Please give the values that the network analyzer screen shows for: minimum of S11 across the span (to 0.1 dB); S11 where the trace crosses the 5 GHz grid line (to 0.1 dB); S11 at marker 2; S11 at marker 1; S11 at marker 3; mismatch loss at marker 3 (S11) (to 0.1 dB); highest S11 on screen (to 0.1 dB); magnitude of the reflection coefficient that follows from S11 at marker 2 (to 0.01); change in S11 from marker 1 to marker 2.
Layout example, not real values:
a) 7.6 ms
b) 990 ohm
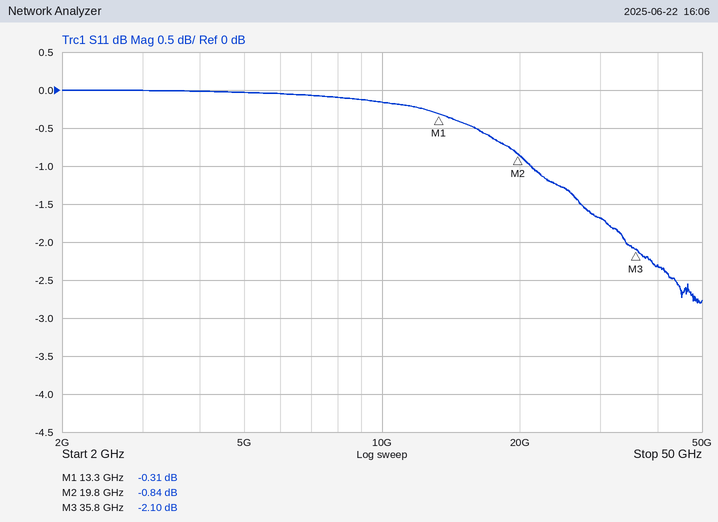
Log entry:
a) -2.8 dB
b) 0.0 dB
c) -0.84 dB
d) -0.31 dB
e) -2.10 dB
f) 4.2 dB
g) 0.0 dB
h) 0.91
i) -0.53 dB
